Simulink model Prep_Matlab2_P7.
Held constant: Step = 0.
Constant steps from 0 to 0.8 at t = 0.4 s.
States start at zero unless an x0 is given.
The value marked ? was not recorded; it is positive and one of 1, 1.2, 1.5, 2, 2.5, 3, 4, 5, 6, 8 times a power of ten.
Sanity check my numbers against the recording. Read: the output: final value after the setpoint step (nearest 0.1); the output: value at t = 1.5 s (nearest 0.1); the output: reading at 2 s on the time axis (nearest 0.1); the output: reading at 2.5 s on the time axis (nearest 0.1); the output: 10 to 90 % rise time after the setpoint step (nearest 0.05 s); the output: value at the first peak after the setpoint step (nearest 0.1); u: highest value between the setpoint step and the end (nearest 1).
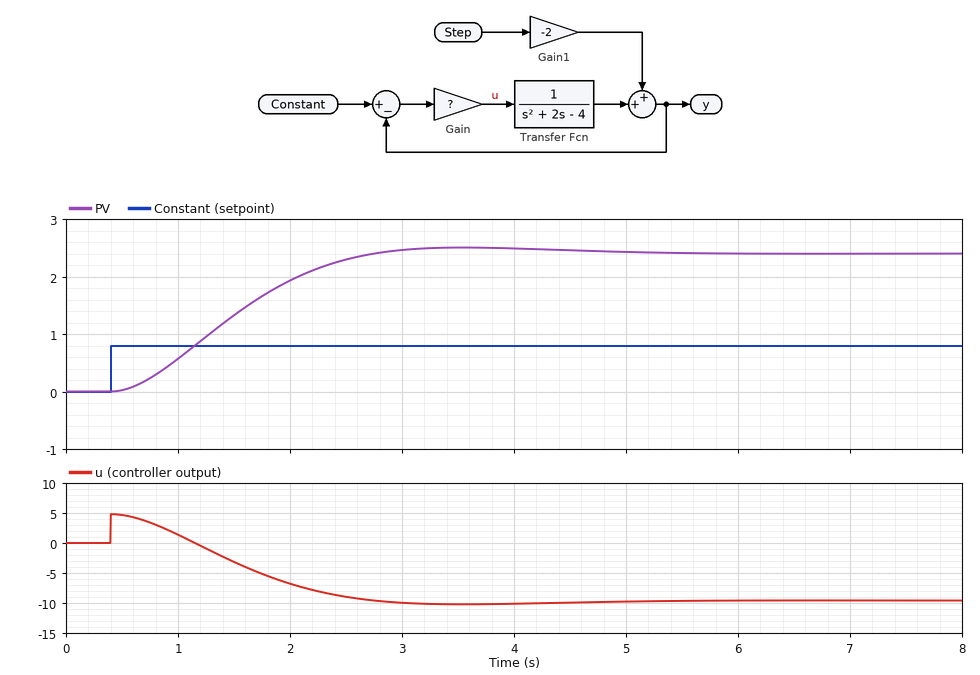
2.4
1.3
1.9
2.3
1.50 s
2.5
5
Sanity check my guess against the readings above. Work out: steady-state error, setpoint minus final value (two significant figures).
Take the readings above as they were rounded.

-1.6
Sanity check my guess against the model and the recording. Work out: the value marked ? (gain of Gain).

6
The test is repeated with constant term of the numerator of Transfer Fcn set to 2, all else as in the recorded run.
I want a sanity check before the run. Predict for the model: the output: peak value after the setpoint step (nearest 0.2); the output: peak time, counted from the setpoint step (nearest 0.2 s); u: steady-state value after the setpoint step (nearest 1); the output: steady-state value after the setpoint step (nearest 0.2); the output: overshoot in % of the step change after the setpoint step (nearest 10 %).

1.6
1.2 s
-2
1.2
30 %
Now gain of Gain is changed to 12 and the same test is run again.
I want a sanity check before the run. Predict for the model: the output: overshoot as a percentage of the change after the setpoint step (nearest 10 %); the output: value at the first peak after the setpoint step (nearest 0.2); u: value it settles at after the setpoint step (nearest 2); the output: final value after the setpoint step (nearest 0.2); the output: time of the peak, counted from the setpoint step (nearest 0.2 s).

30 %
1.6
-4
1.2
1.2 s
